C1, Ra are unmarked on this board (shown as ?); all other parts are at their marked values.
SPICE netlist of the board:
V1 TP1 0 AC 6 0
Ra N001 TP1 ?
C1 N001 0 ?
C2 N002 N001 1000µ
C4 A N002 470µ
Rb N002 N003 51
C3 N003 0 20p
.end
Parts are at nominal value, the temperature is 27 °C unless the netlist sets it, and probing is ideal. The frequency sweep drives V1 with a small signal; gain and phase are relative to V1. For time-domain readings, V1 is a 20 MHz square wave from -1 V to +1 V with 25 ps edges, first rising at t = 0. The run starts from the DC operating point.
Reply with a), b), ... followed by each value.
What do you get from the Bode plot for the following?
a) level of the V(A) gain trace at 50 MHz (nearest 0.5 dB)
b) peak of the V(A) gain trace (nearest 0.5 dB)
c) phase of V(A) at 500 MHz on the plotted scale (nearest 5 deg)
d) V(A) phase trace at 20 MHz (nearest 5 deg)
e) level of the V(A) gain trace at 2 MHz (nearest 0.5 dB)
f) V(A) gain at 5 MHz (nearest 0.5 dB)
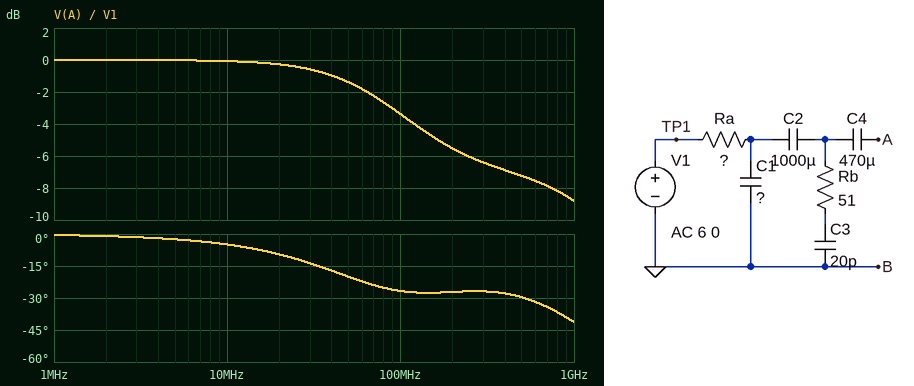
a) -1.5 dB
b) 0 dB
c) -30 deg
d) -10 deg
e) 0 dB
f) 0 dB
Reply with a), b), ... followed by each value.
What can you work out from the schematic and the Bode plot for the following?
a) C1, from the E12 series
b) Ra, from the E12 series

a) 4.7 pF
b) 56 Ω
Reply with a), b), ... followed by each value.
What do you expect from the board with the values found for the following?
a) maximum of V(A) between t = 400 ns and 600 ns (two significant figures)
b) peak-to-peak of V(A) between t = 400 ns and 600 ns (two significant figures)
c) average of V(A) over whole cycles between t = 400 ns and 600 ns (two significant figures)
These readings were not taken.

a) 2.0 V
b) 2.0 V
c) 1.0 V
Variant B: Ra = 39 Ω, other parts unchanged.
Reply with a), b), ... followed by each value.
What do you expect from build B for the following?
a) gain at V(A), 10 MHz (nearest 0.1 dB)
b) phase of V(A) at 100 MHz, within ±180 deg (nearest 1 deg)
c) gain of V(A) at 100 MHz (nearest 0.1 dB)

a) 0 dB
b) -21 deg
c) -2.3 dB
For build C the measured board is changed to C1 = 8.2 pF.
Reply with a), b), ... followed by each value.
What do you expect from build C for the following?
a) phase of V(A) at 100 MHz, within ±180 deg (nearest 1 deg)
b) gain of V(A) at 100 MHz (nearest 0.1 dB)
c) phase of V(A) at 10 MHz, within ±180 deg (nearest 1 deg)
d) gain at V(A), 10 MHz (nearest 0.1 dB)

a) -31 deg
b) -3.7 dB
c) -6 deg
d) -0.1 dB
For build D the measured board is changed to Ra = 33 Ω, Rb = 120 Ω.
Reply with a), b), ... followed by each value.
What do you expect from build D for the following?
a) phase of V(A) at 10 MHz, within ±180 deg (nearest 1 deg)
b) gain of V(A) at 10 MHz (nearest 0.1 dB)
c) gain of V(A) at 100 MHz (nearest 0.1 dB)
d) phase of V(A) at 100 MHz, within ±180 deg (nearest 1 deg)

a) -3 deg
b) -0.1 dB
c) -1.7 dB
d) -11 deg
